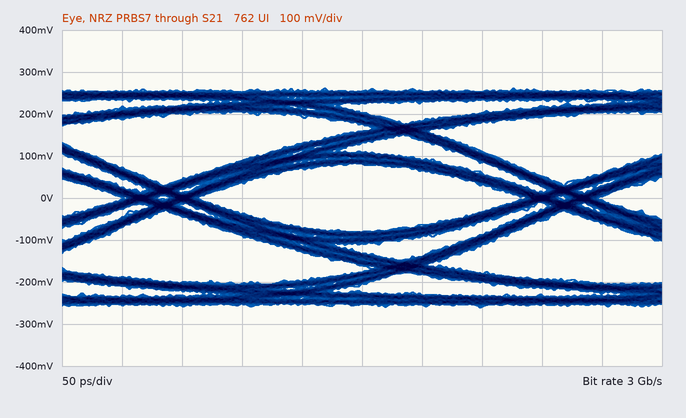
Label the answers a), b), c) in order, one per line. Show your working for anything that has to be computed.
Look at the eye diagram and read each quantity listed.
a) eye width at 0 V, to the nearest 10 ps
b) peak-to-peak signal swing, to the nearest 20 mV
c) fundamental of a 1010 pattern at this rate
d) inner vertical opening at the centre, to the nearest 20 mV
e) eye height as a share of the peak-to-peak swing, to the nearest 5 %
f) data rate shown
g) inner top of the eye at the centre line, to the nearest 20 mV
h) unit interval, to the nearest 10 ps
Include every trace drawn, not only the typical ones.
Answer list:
a) 270 ps
b) 520 mV
c) 1.5 GHz
d) 160 mV
e) 160 mV / 520 mV ≈ 30.8 %, so 30 % to the nearest 5 %
f) 3 Gb/s
g) 80 mV
h) 330 ps
